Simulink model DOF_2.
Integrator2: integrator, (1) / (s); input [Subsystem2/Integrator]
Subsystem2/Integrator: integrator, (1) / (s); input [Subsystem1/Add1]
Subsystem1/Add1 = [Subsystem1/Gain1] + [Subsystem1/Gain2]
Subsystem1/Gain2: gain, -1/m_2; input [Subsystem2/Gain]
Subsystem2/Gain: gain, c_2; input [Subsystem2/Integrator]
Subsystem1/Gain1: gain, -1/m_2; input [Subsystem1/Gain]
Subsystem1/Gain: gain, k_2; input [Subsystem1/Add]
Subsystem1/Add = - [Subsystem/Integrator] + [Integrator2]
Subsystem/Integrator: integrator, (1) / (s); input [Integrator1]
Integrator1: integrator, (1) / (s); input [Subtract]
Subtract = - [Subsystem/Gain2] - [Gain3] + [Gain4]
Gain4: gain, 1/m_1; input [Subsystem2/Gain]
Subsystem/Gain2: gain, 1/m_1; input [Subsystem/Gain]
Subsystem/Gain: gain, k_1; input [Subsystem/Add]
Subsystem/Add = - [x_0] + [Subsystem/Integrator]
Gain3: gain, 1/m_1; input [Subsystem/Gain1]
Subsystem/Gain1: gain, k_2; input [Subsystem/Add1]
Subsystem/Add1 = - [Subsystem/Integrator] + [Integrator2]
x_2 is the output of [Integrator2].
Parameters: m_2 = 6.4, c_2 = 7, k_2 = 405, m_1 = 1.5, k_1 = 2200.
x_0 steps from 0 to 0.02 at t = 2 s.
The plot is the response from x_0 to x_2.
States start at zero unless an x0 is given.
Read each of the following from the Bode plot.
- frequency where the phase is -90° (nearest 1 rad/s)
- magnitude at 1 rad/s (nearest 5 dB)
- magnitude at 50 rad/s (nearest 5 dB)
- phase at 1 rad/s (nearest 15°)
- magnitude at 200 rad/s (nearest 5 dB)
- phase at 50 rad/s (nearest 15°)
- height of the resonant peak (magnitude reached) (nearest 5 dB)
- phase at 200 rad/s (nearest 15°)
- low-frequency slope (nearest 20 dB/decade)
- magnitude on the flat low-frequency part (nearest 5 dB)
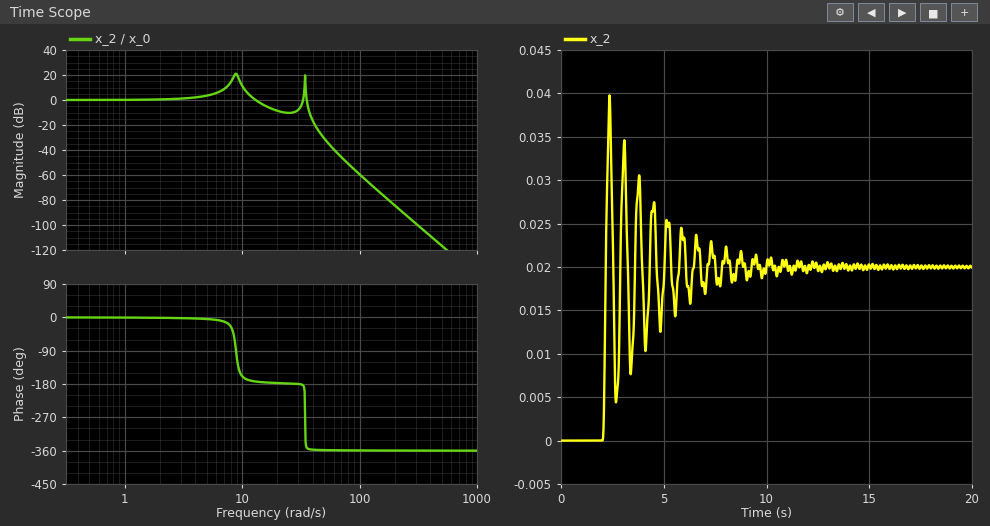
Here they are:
9 rad/s
0 dB
-30 dB
0°
-85 dB
-360°
20 dB
-360°
0 dB/decade
0 dB
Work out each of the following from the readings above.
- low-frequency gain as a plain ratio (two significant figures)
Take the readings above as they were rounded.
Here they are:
1.0
